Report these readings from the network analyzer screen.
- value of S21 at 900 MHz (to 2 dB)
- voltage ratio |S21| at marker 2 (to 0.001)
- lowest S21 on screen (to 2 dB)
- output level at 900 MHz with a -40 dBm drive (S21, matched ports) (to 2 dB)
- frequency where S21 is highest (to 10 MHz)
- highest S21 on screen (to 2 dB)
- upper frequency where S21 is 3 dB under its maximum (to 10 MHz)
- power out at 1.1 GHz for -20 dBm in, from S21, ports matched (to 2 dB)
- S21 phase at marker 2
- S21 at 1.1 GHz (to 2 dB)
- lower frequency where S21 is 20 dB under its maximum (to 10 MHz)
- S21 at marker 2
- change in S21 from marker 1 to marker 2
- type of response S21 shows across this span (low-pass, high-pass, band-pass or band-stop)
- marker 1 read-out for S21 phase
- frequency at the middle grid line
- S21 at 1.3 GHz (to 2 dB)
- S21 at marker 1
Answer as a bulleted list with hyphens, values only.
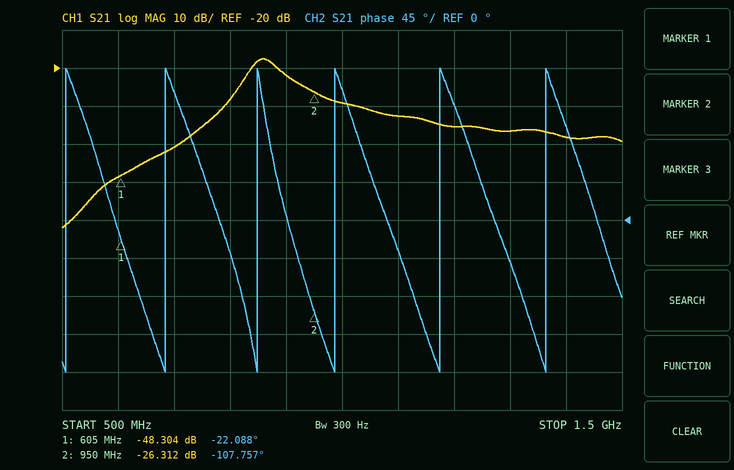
- -22 dB
- 0.048
- -62 dB
- -62 dBm
- 860 MHz
- -18 dB
- 890 MHz
- -52 dBm
- -107.757°
- -32 dB
- 730 MHz
- -26.312 dB
- 21.992 dB
- band-pass
- -22.088°
- 1 GHz
- -36 dB
- -48.304 dB
